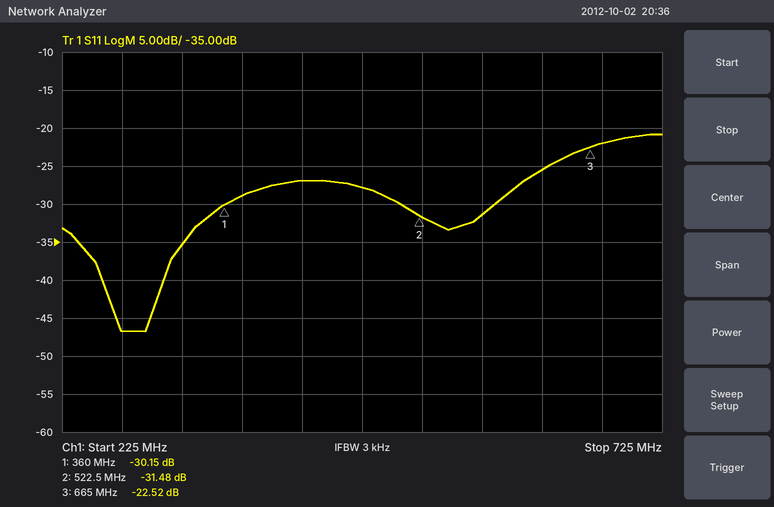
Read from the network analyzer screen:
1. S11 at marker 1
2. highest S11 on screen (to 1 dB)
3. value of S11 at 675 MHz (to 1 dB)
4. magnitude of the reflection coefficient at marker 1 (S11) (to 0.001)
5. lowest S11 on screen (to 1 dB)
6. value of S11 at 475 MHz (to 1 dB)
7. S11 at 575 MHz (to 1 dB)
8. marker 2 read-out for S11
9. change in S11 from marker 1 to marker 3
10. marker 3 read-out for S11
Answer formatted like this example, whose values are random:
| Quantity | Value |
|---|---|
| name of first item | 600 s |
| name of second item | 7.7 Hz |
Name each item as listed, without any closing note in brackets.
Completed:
| Quantity | Value |
|---|---|
| S11 at marker 1 | -30.15 dB |
| highest S11 on screen | -21 dB |
| value of S11 at 675 MHz | -22 dB |
| magnitude of the reflection coefficient at marker 1 (S11) | 0.031 |
| lowest S11 on screen | -47 dB |
| value of S11 at 475 MHz | -28 dB |
| S11 at 575 MHz | -31 dB |
| marker 2 read-out for S11 | -31.48 dB |
| change in S11 from marker 1 to marker 3 | 7.63 dB |
| marker 3 read-out for S11 | -22.52 dB |
